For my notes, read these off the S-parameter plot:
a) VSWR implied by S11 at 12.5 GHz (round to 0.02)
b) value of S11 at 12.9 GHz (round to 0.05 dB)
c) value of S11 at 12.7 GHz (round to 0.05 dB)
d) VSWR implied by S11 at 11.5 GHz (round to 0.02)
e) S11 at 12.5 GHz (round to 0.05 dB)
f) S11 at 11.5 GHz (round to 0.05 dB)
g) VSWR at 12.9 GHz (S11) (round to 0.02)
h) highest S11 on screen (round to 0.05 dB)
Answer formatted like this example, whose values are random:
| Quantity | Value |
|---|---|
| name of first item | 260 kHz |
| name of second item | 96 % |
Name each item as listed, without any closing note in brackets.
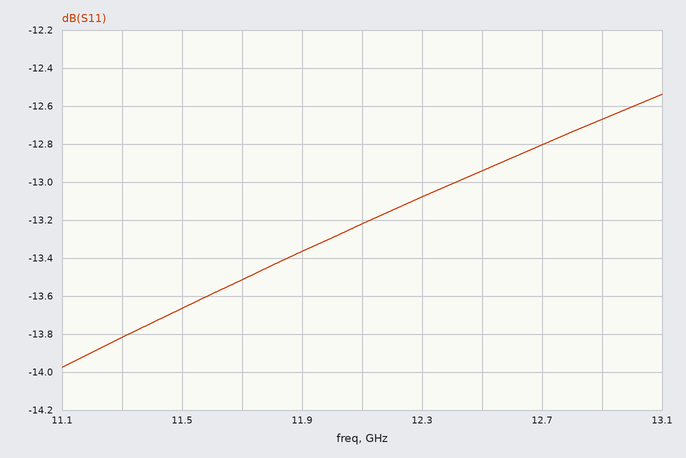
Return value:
| Quantity | Value |
|---|---|
| VSWR implied by S11 at 12.5 GHz | 1.58 |
| value of S11 at 12.9 GHz | -12.65 dB |
| value of S11 at 12.7 GHz | -12.80 dB |
| VSWR implied by S11 at 11.5 GHz | 1.52 |
| S11 at 12.5 GHz | -12.95 dB |
| S11 at 11.5 GHz | -13.65 dB |
| VSWR at 12.9 GHz (S11) | 1.60 |
| highest S11 on screen | -12.55 dB |
